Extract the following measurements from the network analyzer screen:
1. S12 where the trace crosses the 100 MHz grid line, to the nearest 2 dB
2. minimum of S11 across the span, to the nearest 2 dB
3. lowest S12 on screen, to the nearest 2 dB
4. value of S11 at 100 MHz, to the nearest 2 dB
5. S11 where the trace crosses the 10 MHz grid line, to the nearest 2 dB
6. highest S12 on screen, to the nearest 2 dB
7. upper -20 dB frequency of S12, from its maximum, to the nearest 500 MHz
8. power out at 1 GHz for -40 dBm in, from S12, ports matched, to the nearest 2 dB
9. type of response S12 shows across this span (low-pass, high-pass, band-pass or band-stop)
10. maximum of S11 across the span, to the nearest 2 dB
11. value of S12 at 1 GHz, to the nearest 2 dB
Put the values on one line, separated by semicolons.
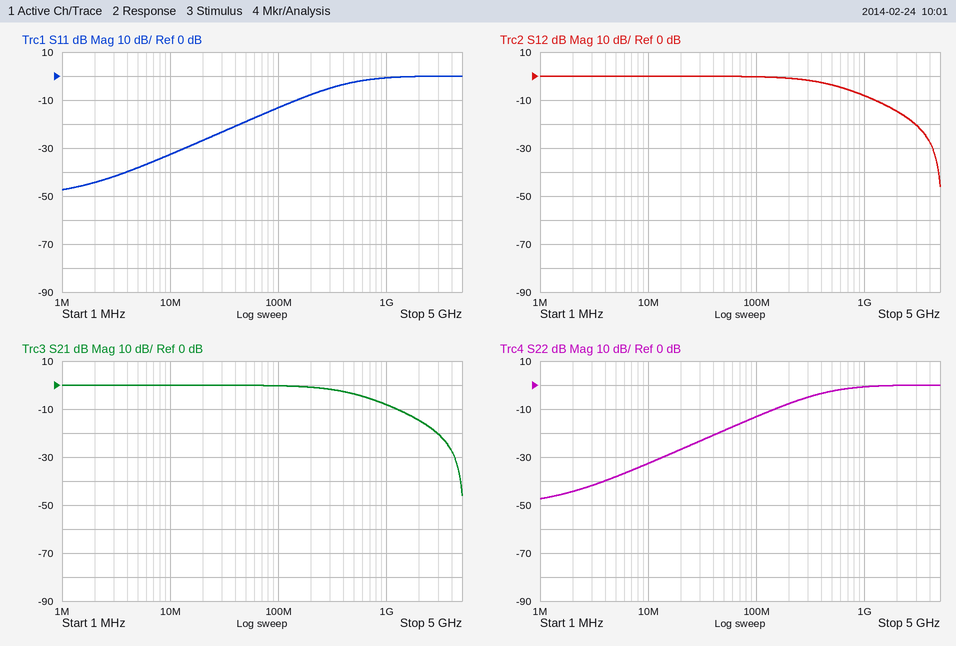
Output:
0 dB; -48 dB; -46 dB; -14 dB; -32 dB; 0 dB; 3.0 GHz; -48 dBm; low-pass; 0 dB; -8 dB
